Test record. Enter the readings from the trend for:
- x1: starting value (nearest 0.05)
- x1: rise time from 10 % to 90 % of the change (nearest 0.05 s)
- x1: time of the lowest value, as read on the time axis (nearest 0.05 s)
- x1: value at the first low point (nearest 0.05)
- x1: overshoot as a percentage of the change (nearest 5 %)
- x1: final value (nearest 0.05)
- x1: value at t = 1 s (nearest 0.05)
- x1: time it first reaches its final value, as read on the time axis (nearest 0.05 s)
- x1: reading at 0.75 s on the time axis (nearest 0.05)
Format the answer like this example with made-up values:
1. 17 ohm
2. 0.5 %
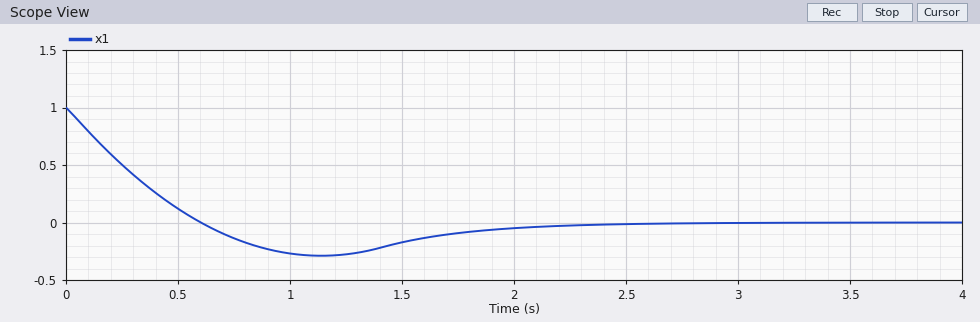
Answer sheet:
1. 1.00
2. 0.45 s
3. 1.15 s
4. -0.30
5. 30 %
6. 0.00
7. -0.25
8. 0.60 s
9. -0.15
